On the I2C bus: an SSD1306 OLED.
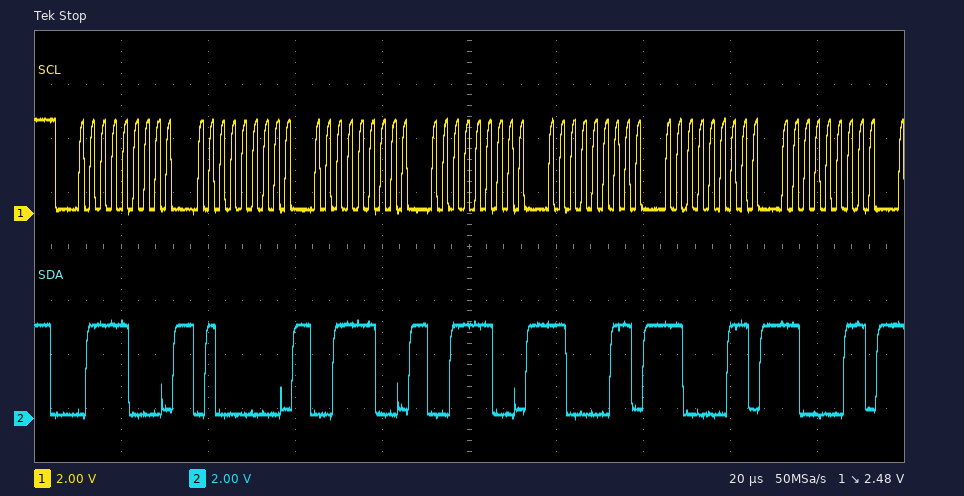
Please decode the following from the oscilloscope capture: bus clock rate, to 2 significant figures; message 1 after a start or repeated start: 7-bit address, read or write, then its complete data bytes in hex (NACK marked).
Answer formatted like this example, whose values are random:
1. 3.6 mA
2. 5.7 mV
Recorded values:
1. 400 kHz
2. 0x3C write: 40 3C 3C C3 C3 C3
